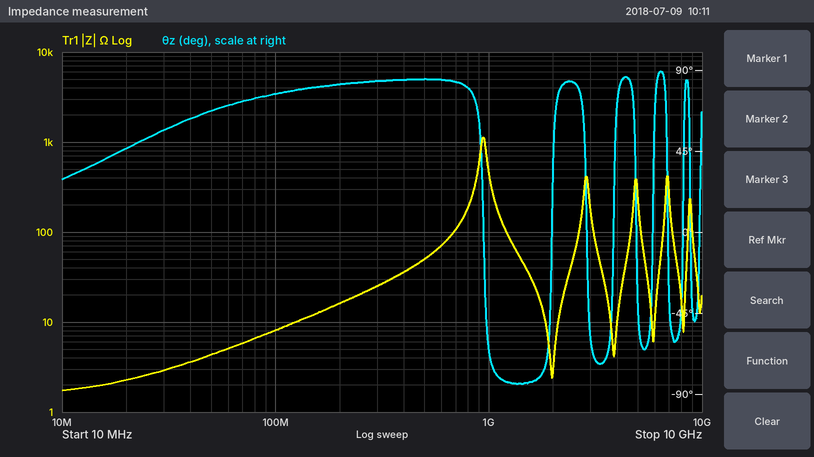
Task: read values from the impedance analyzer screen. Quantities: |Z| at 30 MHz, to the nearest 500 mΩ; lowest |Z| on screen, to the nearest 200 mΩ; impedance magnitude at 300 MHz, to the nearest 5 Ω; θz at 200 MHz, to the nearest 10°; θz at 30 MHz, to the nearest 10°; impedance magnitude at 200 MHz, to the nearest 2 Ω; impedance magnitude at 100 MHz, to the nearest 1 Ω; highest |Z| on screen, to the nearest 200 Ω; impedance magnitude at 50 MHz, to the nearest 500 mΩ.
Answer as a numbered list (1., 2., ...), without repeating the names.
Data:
1. 3.0 Ω
2. 1.8 Ω
3. 25 Ω
4. 80°
5. 60°
6. 16 Ω
7. 8 Ω
8. 1.2 kΩ
9. 4.5 Ω
